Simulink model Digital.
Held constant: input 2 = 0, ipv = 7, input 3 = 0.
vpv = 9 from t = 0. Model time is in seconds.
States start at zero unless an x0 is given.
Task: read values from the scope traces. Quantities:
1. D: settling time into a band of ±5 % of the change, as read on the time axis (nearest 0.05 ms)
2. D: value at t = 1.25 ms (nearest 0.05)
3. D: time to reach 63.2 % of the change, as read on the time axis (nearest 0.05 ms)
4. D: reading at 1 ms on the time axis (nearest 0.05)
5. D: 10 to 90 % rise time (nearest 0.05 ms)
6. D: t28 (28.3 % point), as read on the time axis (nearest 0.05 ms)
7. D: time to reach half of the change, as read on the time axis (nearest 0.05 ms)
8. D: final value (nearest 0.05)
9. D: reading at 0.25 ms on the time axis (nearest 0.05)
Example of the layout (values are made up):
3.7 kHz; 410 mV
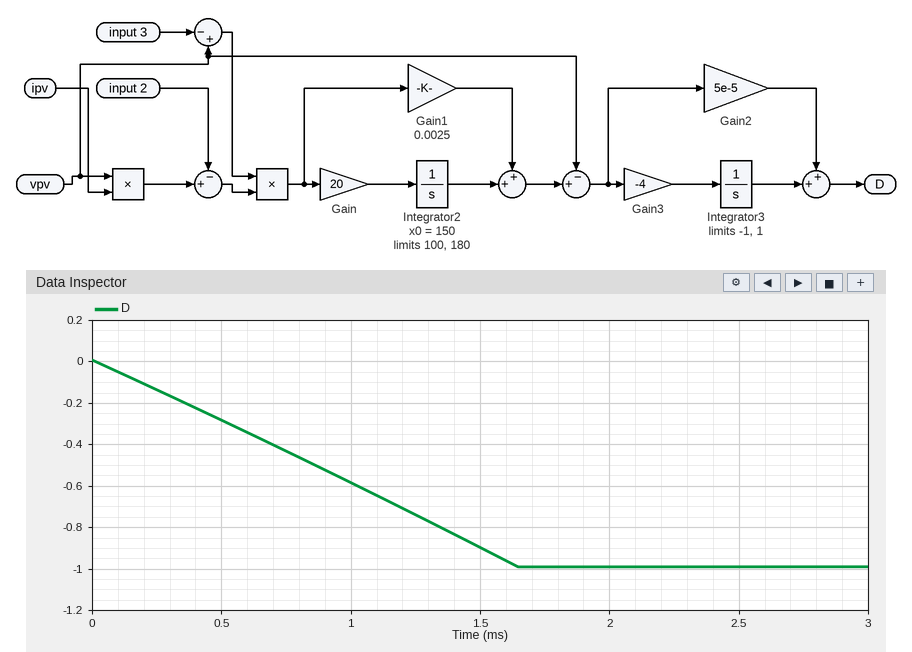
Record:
1.55 ms; -0.75; 1.05 ms; -0.60; 1.30 ms; 0.50 ms; 0.85 ms; -1.00; -0.15
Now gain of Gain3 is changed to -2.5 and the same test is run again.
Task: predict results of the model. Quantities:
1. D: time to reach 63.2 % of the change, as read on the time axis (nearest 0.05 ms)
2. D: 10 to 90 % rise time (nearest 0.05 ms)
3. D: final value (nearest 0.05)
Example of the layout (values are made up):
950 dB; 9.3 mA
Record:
1.65 ms; 2.05 ms; -1.00
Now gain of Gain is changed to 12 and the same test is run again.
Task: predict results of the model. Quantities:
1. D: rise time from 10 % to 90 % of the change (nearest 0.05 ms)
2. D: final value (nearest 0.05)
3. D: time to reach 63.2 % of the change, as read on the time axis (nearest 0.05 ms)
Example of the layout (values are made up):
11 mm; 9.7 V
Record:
1.35 ms; -1.00; 1.10 ms
